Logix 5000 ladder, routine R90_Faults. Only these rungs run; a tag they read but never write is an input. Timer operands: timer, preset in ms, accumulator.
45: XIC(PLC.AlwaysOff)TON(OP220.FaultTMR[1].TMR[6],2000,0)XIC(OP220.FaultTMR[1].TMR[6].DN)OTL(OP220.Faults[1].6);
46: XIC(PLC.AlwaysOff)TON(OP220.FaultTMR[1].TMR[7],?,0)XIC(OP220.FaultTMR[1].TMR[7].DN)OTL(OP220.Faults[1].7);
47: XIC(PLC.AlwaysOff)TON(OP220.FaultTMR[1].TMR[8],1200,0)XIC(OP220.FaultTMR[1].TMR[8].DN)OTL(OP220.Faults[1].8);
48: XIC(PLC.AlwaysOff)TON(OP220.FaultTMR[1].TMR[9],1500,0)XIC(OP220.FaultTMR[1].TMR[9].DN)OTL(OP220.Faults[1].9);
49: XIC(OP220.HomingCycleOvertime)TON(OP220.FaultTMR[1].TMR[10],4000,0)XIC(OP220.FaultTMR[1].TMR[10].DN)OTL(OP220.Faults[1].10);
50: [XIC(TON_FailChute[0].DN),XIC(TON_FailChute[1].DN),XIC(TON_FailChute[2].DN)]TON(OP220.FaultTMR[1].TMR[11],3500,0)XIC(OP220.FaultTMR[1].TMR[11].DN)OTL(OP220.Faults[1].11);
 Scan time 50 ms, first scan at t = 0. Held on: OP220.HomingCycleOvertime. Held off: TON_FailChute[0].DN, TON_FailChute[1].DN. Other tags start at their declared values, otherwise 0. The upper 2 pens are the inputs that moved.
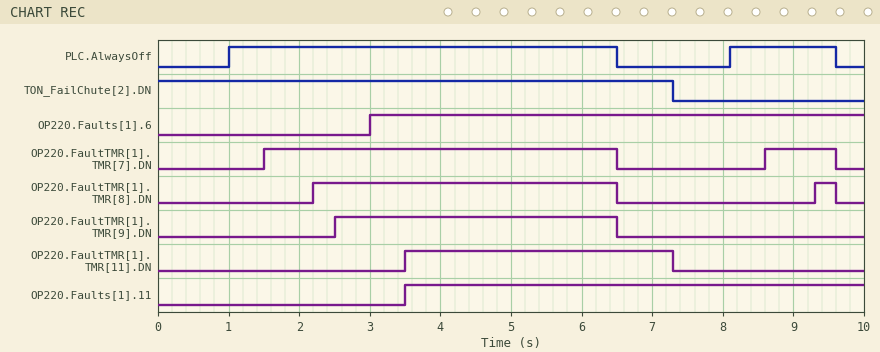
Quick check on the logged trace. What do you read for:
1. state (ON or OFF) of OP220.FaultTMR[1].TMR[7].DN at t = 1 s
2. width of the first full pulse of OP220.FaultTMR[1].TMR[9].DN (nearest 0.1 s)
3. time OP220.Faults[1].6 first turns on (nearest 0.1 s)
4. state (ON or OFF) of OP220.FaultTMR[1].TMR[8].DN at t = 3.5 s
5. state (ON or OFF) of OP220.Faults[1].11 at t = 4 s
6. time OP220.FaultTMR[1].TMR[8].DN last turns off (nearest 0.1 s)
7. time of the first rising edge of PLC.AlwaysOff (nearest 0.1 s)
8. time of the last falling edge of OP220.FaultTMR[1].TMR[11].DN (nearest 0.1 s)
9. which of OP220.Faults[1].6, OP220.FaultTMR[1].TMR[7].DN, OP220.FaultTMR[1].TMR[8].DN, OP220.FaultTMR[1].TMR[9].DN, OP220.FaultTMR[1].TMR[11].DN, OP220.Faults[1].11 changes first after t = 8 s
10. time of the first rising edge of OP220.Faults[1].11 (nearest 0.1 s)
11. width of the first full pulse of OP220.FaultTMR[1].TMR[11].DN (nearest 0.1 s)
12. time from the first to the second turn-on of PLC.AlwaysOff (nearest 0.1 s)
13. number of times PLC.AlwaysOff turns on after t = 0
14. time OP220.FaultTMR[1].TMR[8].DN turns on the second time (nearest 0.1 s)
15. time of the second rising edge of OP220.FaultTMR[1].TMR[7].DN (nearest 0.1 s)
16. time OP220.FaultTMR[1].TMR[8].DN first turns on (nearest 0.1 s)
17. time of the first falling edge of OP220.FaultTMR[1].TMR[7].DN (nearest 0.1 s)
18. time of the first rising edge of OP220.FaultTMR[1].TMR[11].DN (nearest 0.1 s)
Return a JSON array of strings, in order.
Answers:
["OFF", "4.0 s", "3.0 s", "ON", "ON", "9.6 s", "1.0 s", "7.3 s", "OP220.FaultTMR[1].TMR[7].DN", "3.5 s", "3.8 s", "7.1 s", "2", "9.3 s", "8.6 s", "2.2 s", "6.5 s", "3.5 s"]
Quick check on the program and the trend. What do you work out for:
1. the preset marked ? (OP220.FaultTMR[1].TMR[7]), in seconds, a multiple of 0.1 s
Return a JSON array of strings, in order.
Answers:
["0.5 s"]
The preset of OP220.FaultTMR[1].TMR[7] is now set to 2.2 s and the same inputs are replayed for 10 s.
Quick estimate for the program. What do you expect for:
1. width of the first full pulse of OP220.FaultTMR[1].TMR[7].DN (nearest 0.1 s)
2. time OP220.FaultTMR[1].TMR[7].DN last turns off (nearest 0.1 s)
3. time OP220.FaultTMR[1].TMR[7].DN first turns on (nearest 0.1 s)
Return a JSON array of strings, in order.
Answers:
["3.3 s", "6.5 s", "3.2 s"]
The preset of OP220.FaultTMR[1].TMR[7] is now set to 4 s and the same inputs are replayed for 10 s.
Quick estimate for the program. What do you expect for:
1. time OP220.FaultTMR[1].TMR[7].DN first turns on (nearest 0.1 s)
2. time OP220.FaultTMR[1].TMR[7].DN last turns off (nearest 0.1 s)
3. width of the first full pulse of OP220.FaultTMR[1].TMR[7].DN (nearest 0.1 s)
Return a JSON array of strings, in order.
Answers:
["5.0 s", "6.5 s", "1.5 s"]
